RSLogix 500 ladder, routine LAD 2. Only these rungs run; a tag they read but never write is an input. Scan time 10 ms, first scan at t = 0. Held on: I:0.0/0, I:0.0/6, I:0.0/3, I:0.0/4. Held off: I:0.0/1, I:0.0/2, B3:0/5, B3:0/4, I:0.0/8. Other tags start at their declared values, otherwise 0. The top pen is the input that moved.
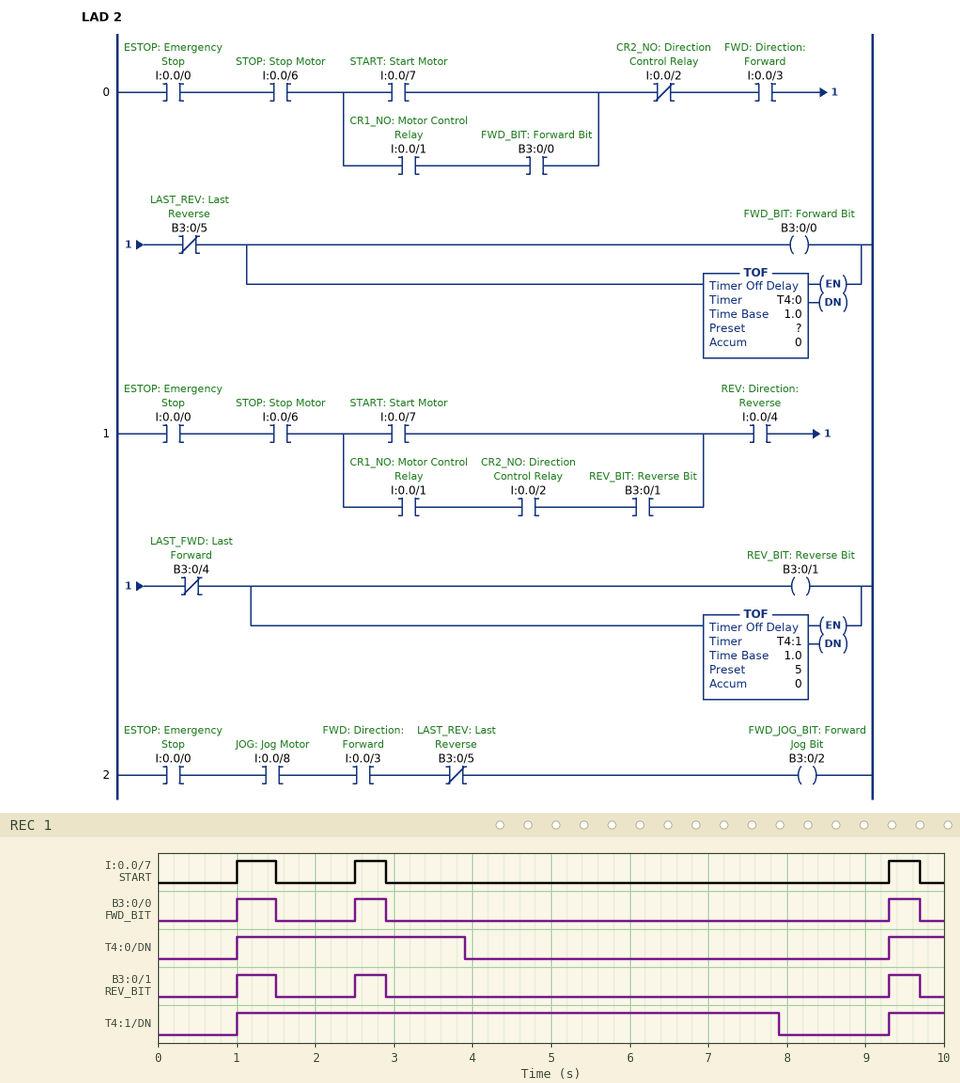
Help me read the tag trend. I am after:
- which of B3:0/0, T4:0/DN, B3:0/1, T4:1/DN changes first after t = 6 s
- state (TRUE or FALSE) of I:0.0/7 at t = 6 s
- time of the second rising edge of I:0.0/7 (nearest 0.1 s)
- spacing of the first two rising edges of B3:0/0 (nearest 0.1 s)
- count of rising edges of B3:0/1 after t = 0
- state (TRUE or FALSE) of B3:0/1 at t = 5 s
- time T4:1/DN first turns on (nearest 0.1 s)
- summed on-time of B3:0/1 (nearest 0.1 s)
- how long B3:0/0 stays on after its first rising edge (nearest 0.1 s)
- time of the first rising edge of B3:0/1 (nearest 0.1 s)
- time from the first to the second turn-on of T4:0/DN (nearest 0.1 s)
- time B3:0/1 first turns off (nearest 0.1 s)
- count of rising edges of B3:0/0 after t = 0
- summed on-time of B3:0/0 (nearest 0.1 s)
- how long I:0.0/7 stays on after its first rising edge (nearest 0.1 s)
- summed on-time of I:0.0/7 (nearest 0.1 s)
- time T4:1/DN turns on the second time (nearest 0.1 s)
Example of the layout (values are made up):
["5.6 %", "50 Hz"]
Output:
["T4:1/DN", "FALSE", "2.5 s", "1.5 s", "3", "FALSE", "1.0 s", "1.3 s", "0.5 s", "1.0 s", "8.3 s", "1.5 s", "3", "1.3 s", "0.5 s", "1.3 s", "9.3 s"]
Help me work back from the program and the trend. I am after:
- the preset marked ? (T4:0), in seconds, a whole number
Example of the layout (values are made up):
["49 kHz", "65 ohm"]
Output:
["1 s"]
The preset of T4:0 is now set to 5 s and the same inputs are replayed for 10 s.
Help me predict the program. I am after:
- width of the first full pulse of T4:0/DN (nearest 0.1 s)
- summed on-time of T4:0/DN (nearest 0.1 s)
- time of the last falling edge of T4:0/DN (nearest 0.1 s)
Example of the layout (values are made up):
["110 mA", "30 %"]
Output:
["6.9 s", "7.6 s", "7.9 s"]
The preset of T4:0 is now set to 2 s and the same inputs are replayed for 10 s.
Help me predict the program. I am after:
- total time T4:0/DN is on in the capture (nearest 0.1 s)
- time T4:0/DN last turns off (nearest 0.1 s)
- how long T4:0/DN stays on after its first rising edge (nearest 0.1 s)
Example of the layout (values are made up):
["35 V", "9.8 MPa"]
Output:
["4.6 s", "4.9 s", "3.9 s"]
